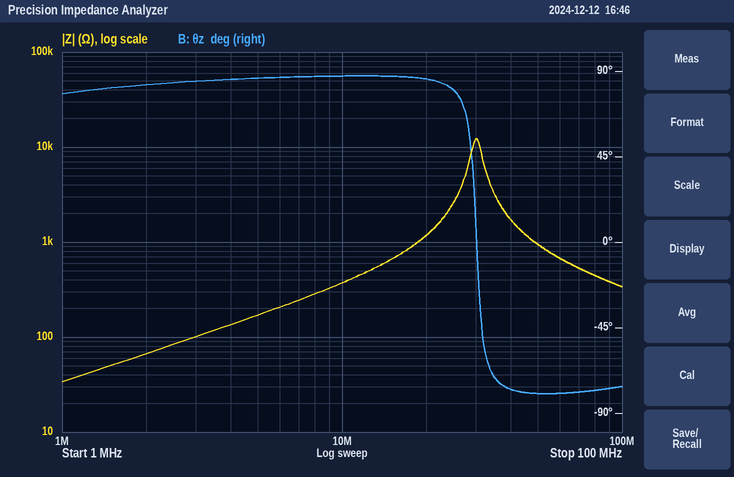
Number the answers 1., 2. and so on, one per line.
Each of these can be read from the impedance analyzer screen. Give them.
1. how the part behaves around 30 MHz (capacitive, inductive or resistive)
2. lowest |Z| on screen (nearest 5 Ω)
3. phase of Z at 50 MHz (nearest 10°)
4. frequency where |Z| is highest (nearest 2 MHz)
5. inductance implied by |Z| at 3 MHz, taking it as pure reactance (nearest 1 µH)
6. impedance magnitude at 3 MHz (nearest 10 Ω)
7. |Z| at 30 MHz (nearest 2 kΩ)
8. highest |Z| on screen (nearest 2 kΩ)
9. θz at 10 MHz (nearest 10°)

1. resistive
2. 35 Ω
3. -80°
4. 30 MHz
5. 5 µH
6. 100 Ω
7. 12 kΩ
8. 12 kΩ
9. 90°
